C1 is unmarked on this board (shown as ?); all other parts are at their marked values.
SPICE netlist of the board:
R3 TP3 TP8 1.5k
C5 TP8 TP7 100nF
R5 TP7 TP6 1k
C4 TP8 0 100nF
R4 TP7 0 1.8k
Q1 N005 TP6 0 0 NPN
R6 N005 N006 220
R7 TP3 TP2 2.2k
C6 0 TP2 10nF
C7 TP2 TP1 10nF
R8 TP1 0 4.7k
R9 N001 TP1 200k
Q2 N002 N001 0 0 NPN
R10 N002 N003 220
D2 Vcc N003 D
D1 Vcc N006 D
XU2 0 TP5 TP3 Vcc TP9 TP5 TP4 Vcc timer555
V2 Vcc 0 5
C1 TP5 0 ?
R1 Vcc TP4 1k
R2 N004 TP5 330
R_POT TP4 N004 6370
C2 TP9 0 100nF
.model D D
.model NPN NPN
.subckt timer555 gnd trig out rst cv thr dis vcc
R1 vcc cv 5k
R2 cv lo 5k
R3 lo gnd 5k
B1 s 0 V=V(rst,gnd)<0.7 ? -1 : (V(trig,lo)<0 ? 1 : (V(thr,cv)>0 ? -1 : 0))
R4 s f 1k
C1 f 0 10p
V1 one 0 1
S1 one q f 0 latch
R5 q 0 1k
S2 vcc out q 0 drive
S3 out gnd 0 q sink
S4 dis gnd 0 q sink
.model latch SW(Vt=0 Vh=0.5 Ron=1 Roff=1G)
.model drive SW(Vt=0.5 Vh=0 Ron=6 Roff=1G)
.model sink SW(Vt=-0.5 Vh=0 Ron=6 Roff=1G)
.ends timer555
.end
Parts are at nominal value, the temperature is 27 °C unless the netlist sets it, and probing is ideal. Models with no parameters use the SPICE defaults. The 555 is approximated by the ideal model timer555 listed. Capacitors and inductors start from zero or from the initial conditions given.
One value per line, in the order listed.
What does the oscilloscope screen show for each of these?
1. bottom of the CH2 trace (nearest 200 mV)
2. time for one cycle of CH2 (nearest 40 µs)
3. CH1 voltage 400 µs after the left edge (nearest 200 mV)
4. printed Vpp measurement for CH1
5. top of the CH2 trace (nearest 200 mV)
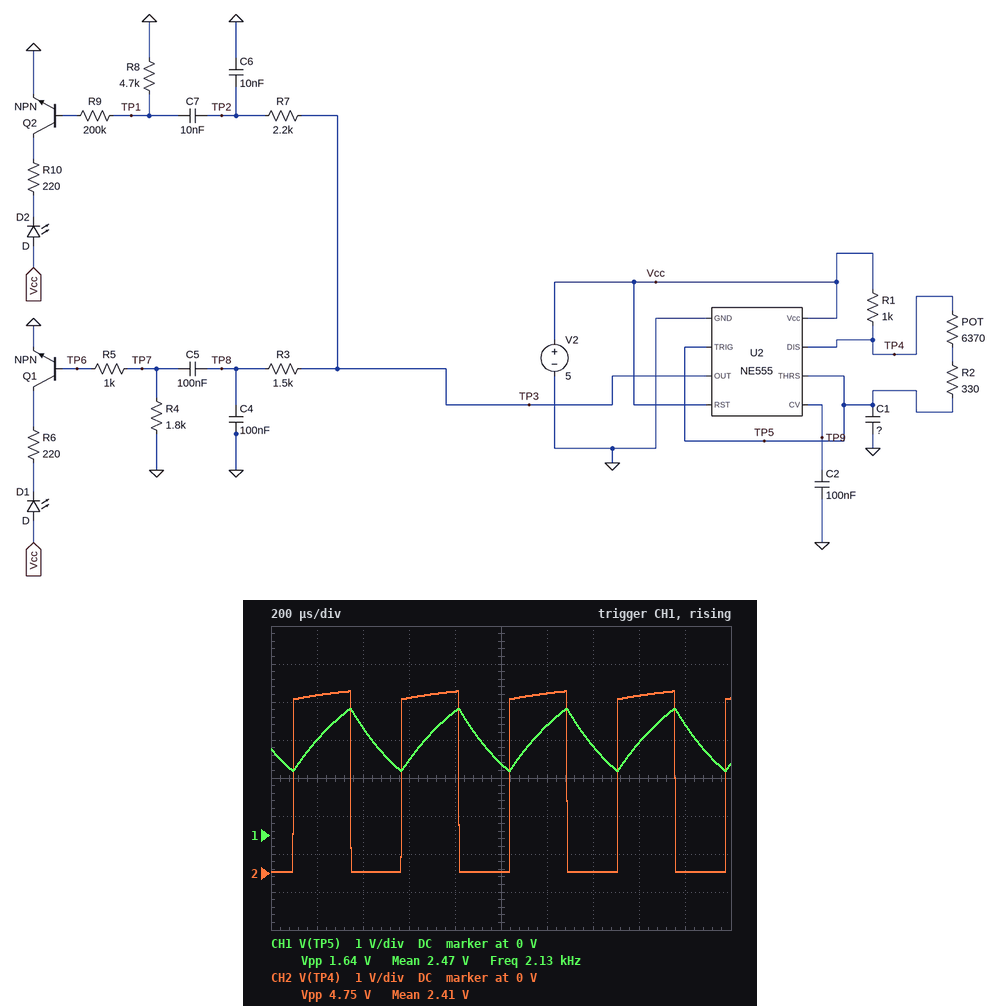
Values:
0 V
480 µs
2.8 V
1.64 V
4.8 V
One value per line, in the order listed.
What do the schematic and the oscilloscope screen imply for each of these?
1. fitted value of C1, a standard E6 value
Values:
47 nF
